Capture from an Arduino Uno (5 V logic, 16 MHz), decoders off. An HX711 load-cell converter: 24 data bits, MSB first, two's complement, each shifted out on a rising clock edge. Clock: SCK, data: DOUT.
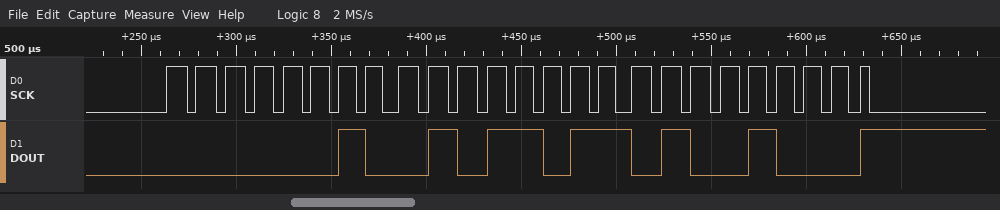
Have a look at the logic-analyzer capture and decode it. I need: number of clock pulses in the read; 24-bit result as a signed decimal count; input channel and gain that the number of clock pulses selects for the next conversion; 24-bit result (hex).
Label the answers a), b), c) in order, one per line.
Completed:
a) 25
b) 154440
c) channel A, gain 128
d) 0x025B48
